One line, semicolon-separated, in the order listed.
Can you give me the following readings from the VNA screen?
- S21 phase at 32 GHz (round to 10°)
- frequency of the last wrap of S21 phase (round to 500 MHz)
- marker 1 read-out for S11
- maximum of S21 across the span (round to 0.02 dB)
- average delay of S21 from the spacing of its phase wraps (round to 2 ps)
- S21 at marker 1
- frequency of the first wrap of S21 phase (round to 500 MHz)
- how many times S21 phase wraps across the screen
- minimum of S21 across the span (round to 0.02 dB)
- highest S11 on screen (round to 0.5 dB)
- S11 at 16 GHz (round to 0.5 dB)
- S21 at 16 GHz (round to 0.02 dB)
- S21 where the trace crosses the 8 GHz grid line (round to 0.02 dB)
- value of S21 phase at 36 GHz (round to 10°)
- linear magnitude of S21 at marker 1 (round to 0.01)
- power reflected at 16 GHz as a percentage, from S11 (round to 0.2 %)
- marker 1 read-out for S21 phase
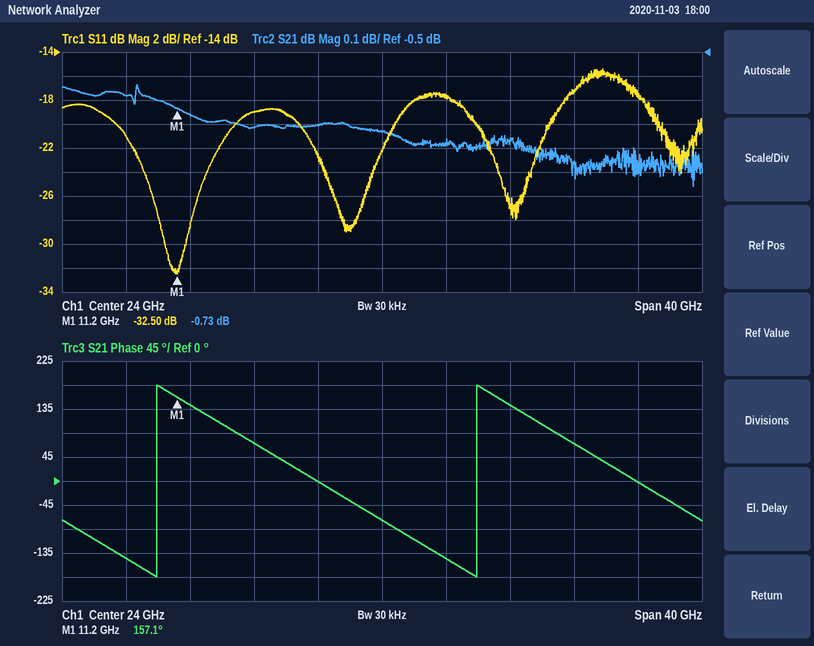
140°; 30.0 GHz; -32.50 dB; -0.64 dB; 50 ps; -0.73 dB; 10.0 GHz; 2; -1.06 dB; -15.5 dB; -19.0 dB; -0.82 dB; -0.68 dB; 70°; 0.92; 1.2 %; 157.1°
